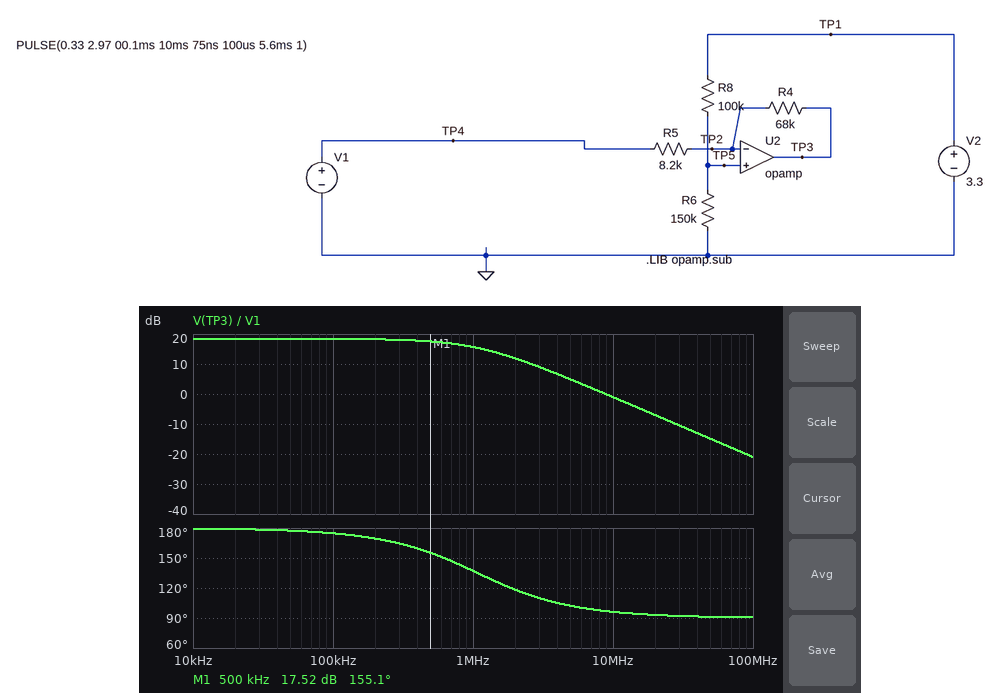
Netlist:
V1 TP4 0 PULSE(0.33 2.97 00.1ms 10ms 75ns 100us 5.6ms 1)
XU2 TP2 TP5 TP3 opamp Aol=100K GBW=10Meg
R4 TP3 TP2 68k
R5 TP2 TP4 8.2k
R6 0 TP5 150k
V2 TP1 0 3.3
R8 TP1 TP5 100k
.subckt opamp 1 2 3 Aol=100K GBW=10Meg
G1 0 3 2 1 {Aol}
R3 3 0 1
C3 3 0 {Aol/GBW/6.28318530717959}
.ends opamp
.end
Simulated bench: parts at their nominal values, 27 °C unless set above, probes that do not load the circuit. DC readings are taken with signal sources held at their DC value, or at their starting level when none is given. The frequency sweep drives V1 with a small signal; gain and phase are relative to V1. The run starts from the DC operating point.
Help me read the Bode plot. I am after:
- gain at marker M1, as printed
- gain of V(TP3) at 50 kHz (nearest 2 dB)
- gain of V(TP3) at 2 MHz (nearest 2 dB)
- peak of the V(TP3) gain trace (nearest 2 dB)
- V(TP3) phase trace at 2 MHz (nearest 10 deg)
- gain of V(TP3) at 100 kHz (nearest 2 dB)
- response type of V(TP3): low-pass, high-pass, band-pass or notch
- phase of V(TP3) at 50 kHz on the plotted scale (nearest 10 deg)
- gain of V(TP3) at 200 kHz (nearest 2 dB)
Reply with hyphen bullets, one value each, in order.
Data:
- 17.52 dB
- 18 dB
- 12 dB
- 18 dB
- 120 deg
- 18 dB
- low-pass
- 180 deg
- 18 dB
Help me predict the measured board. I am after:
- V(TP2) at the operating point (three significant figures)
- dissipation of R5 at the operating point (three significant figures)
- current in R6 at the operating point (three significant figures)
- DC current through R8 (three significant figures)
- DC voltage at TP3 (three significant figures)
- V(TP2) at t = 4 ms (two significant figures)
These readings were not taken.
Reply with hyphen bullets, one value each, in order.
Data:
- 1.98 V
- 332 µW
- 13.2 µA
- 13.2 µA
- 15.7 V
- 2.0 V
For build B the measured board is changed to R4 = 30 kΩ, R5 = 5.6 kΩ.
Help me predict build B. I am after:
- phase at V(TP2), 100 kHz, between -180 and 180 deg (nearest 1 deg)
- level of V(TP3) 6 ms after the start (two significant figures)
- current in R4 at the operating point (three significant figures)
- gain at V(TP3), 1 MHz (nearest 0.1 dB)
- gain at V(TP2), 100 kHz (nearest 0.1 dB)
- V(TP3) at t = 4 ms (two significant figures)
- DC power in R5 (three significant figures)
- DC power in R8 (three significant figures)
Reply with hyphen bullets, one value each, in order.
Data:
- 86 deg
- 11 V
- 295 µA
- 13.1 dB
- -25.4 dB
- 5.3 V
- 486 µW
- 17.4 µW
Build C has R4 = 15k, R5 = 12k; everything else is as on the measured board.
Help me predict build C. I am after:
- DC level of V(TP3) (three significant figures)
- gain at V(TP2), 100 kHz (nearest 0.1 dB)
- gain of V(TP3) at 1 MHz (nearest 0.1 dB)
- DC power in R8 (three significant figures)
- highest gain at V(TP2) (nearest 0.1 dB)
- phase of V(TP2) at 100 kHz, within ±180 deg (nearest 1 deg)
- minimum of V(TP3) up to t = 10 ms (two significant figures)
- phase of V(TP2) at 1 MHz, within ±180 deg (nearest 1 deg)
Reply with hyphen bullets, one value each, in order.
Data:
- 4.04 V
- -38.1 dB
- 1.7 dB
- 17.4 µW
- -5.1 dB
- 89 deg
- 2.2 V
- 77 deg
